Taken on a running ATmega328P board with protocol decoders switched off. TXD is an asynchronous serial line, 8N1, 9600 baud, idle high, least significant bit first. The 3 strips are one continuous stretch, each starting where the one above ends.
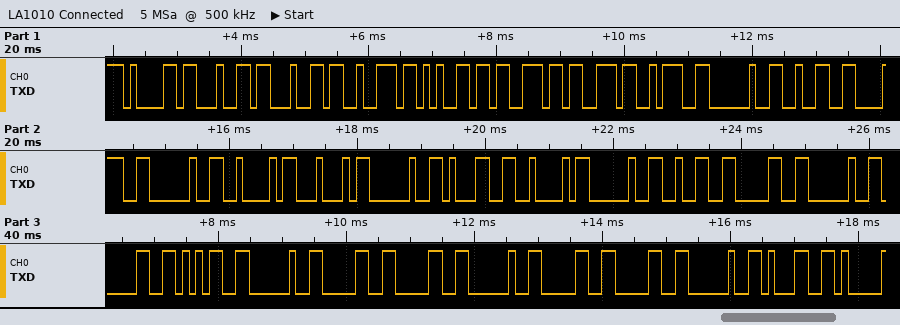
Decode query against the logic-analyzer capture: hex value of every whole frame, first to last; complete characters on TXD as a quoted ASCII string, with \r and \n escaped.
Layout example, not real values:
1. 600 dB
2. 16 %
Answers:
1. 61 64 64 72 65 73 73 3A 20 32 38 20 42 44 20 31 42 20 32 30 20 30 35 20 30 30 20 30 30 20 31
2. "address: 28 BD 1B 20 05 00 00 1"
